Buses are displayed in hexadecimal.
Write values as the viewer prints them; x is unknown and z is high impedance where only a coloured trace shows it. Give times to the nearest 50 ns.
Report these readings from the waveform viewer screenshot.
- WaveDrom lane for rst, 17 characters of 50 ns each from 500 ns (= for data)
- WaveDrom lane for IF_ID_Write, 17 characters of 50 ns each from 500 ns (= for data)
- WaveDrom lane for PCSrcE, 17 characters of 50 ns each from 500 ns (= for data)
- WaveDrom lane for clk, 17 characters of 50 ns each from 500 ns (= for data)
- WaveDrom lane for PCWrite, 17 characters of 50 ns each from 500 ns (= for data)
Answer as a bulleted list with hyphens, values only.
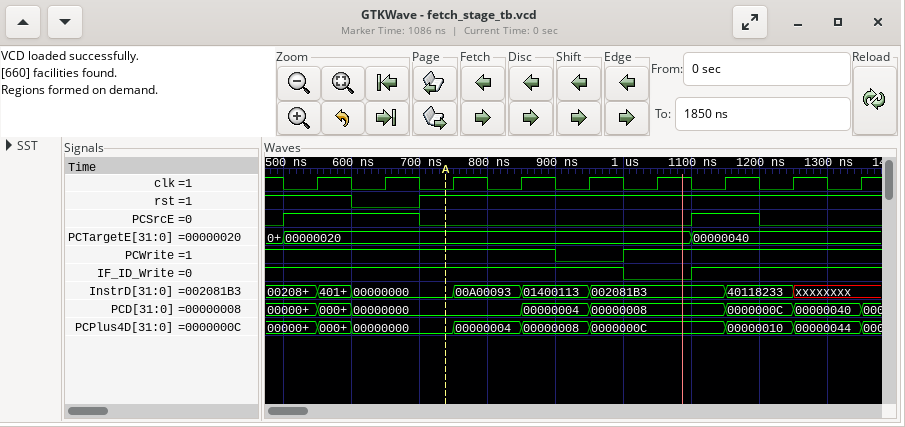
- {name: 'rst', wave: '1.0.1............'}
- {name: 'IF_ID_Write', wave: '1.........0.1....'}
- {name: 'PCSrcE', wave: '1...0.......1.0..'}
- {name: 'clk', wave: '01010101010101010'}
- {name: 'PCWrite', wave: '1.......0.1......'}
